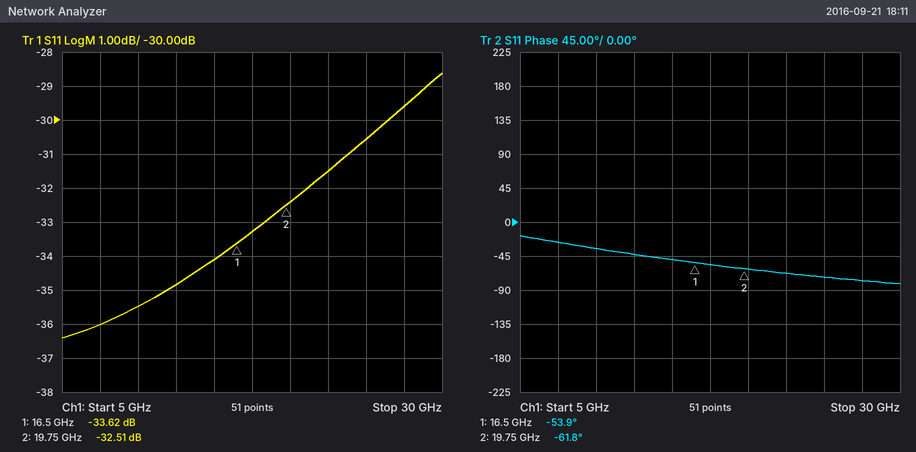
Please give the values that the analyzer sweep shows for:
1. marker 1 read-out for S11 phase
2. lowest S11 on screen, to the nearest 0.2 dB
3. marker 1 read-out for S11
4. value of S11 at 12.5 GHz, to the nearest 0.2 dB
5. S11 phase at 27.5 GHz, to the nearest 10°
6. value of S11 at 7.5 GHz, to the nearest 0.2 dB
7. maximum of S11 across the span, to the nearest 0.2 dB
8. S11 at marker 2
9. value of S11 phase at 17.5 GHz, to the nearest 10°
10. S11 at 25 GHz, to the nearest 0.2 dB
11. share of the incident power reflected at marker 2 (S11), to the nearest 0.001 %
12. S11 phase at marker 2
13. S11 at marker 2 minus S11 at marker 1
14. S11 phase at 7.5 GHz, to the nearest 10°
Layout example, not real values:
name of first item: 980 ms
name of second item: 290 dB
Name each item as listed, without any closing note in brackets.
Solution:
marker 1 read-out for S11 phase: -53.9°
lowest S11 on screen, to the nearest 0.2 dB: -36.4 dB
marker 1 read-out for S11: -33.62 dB
value of S11 at 12.5 GHz, to the nearest 0.2 dB: -34.8 dB
S11 phase at 27.5 GHz, to the nearest 10°: -80°
value of S11 at 7.5 GHz, to the nearest 0.2 dB: -36.0 dB
maximum of S11 across the span, to the nearest 0.2 dB: -28.6 dB
S11 at marker 2: -32.51 dB
value of S11 phase at 17.5 GHz, to the nearest 10°: -60°
S11 at 25 GHz, to the nearest 0.2 dB: -30.6 dB
share of the incident power reflected at marker 2 (S11), to the nearest 0.001 %: 0.056 %
S11 phase at marker 2: -61.8°
S11 at marker 2 minus S11 at marker 1: 1.11 dB
S11 phase at 7.5 GHz, to the nearest 10°: -30°
